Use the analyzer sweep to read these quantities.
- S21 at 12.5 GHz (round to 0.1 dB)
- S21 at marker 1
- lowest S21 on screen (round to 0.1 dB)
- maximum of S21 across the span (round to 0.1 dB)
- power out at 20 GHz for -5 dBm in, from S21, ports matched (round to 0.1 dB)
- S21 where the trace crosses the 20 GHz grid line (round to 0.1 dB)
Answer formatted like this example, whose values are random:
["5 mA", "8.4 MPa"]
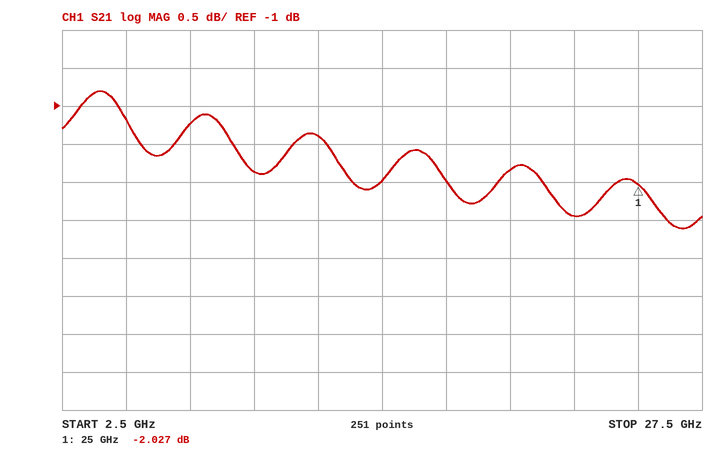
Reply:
["-1.4 dB", "-2.027 dB", "-2.6 dB", "-0.8 dB", "-6.8 dBm", "-1.8 dB"]
